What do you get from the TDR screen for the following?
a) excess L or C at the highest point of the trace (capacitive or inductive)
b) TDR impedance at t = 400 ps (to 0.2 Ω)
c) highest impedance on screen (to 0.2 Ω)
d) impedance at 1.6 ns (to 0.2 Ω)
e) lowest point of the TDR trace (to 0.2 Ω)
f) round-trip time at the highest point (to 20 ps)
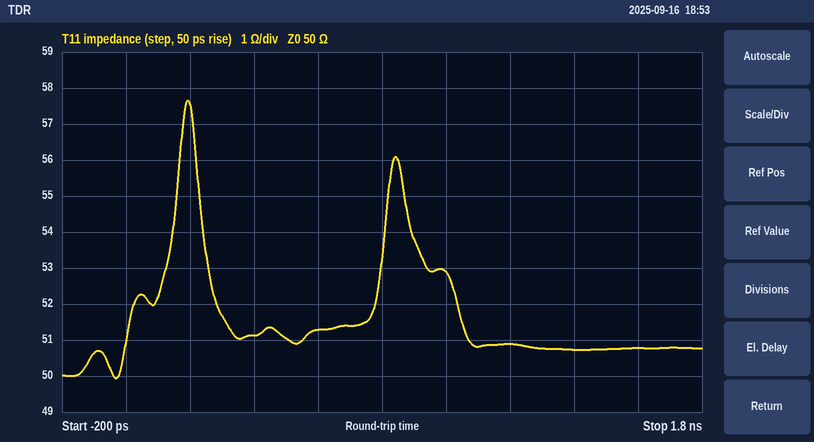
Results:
inductive
51.2 Ω
57.6 Ω
50.8 Ω
50.0 Ω
200 ps
